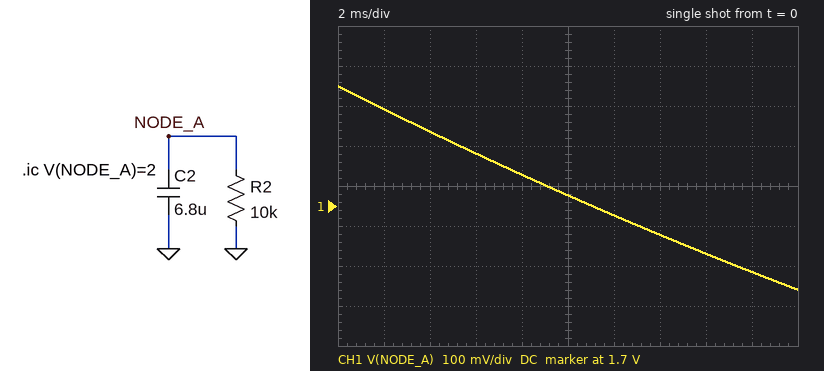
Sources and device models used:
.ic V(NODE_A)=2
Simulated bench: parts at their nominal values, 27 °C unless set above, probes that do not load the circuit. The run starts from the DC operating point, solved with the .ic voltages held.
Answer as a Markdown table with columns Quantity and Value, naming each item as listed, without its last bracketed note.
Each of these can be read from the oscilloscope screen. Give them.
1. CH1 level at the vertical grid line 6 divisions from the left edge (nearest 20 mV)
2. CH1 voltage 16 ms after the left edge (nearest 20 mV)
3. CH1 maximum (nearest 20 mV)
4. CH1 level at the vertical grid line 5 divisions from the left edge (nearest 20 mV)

| Quantity | Value |
|---|---|
| CH1 level at the vertical grid line 6 divisions from the left edge | 1.68 V |
| CH1 voltage 16 ms after the left edge | 1.58 V |
| CH1 maximum | 2.00 V |
| CH1 level at the vertical grid line 5 divisions from the left edge | 1.72 V |
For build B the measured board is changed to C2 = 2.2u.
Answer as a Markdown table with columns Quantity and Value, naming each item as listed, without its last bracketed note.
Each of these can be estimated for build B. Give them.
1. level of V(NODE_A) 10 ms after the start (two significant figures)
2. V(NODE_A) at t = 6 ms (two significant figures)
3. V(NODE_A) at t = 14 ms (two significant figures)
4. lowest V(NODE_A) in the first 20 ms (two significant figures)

| Quantity | Value |
|---|---|
| level of V(NODE_A) 10 ms after the start | 1.3 V |
| V(NODE_A) at t = 6 ms | 1.5 V |
| V(NODE_A) at t = 14 ms | 1.1 V |
| lowest V(NODE_A) in the first 20 ms | 810 mV |
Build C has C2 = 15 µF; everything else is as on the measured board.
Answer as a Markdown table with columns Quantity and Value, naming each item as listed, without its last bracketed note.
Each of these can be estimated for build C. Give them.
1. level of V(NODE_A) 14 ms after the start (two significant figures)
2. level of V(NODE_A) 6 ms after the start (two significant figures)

| Quantity | Value |
|---|---|
| level of V(NODE_A) 14 ms after the start | 1.8 V |
| level of V(NODE_A) 6 ms after the start | 1.9 V |
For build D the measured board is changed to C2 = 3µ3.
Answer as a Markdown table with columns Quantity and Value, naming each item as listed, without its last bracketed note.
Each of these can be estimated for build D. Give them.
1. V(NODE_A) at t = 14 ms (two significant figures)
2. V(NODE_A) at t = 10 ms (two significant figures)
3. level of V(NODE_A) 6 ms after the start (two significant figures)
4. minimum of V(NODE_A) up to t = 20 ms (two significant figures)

| Quantity | Value |
|---|---|
| V(NODE_A) at t = 14 ms | 1.3 V |
| V(NODE_A) at t = 10 ms | 1.5 V |
| level of V(NODE_A) 6 ms after the start | 1.7 V |
| minimum of V(NODE_A) up to t = 20 ms | 1.1 V |
